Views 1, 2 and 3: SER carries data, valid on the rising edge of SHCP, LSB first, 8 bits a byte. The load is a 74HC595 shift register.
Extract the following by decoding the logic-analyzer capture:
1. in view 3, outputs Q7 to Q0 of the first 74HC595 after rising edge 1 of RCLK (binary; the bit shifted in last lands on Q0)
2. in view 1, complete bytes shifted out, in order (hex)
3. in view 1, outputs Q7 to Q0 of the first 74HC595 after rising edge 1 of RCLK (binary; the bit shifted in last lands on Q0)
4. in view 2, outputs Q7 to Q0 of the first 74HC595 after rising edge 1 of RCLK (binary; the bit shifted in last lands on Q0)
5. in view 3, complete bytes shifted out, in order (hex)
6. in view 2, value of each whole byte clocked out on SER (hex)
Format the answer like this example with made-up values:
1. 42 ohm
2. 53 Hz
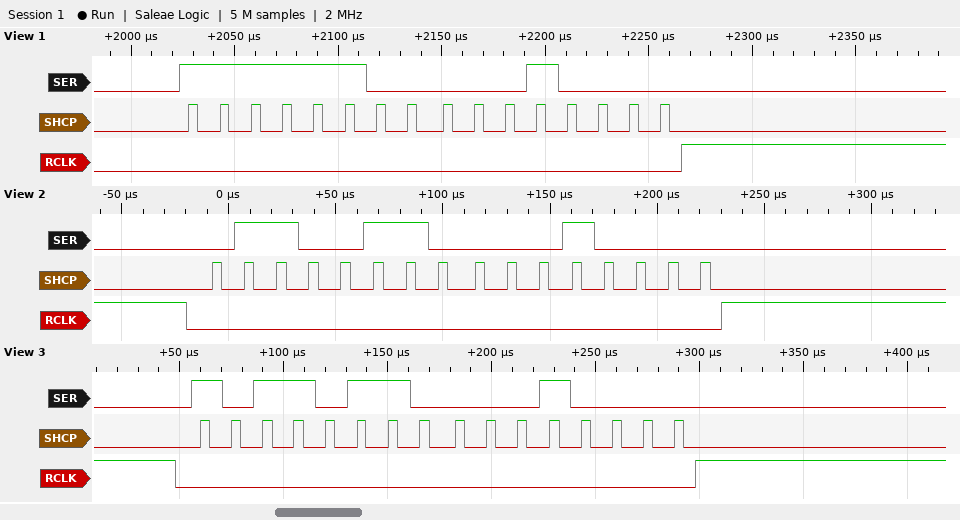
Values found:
1. 00010000
2. 3F 08
3. 00010000
4. 00010000
5. 6D 08
6. 66 08
